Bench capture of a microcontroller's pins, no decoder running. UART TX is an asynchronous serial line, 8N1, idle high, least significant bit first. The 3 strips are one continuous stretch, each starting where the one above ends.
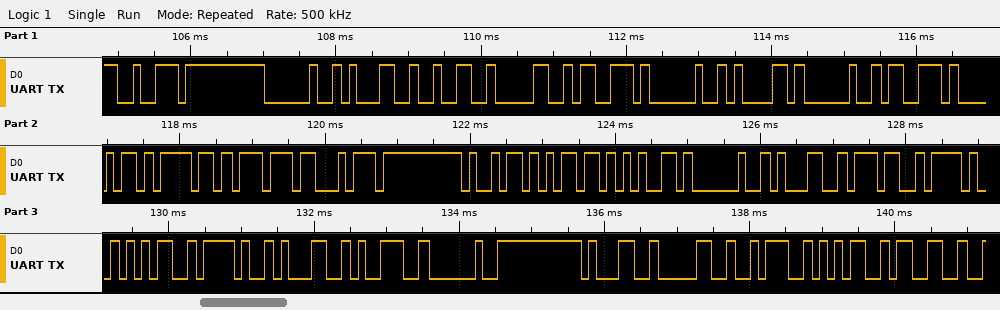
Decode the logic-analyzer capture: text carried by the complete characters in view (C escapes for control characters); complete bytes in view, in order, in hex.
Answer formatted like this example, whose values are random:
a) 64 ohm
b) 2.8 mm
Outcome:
a) "r 120s a showtime 17/5/19 10:53"
b) 72 20 31 32 30 73 20 61 20 73 68 6F 77 74 69 6D 65 20 31 37 2F 35 2F 31 39 20 31 30 3A 35 33
